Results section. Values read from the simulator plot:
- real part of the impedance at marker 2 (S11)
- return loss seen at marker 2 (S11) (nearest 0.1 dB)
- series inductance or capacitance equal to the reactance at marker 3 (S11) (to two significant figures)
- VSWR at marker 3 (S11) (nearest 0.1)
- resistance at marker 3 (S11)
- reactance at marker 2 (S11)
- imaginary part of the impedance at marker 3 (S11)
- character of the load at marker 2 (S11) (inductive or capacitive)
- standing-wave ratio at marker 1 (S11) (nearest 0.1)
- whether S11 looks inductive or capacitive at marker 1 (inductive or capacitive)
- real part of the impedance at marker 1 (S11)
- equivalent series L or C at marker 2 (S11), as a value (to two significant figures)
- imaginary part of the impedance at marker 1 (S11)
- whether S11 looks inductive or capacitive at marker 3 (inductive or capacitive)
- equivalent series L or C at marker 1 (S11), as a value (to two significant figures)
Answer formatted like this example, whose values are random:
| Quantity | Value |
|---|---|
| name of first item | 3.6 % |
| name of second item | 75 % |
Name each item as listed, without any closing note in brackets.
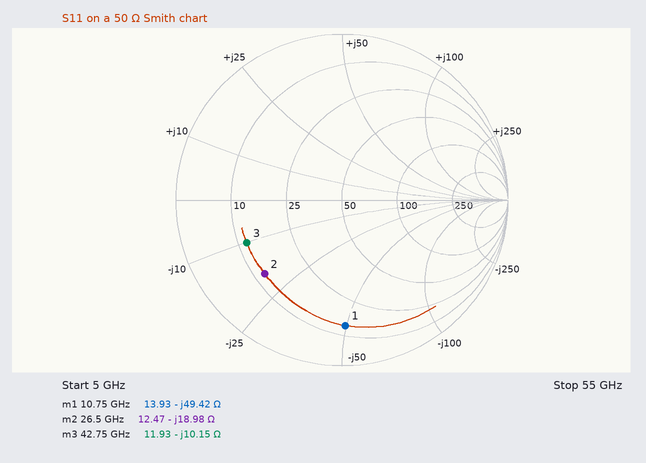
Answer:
| Quantity | Value |
|---|---|
| real part of the impedance at marker 2 | 12.47 Ω |
| return loss seen at marker 2 (S11) | 3.8 dB |
| series inductance or capacitance equal to the reactance at marker 3 (S11) | 370 fF |
| VSWR at marker 3 (S11) | 4.4 |
| resistance at marker 3 | 11.93 Ω |
| reactance at marker 2 | -18.98 Ω |
| imaginary part of the impedance at marker 3 | -10.15 Ω |
| character of the load at marker 2 (S11) | capacitive |
| standing-wave ratio at marker 1 (S11) | 7.2 |
| whether S11 looks inductive or capacitive at marker 1 | capacitive |
| real part of the impedance at marker 1 | 13.93 Ω |
| equivalent series L or C at marker 2 (S11), as a value | 320 fF |
| imaginary part of the impedance at marker 1 | -49.42 Ω |
| whether S11 looks inductive or capacitive at marker 3 | capacitive |
| equivalent series L or C at marker 1 (S11), as a value | 300 fF |
